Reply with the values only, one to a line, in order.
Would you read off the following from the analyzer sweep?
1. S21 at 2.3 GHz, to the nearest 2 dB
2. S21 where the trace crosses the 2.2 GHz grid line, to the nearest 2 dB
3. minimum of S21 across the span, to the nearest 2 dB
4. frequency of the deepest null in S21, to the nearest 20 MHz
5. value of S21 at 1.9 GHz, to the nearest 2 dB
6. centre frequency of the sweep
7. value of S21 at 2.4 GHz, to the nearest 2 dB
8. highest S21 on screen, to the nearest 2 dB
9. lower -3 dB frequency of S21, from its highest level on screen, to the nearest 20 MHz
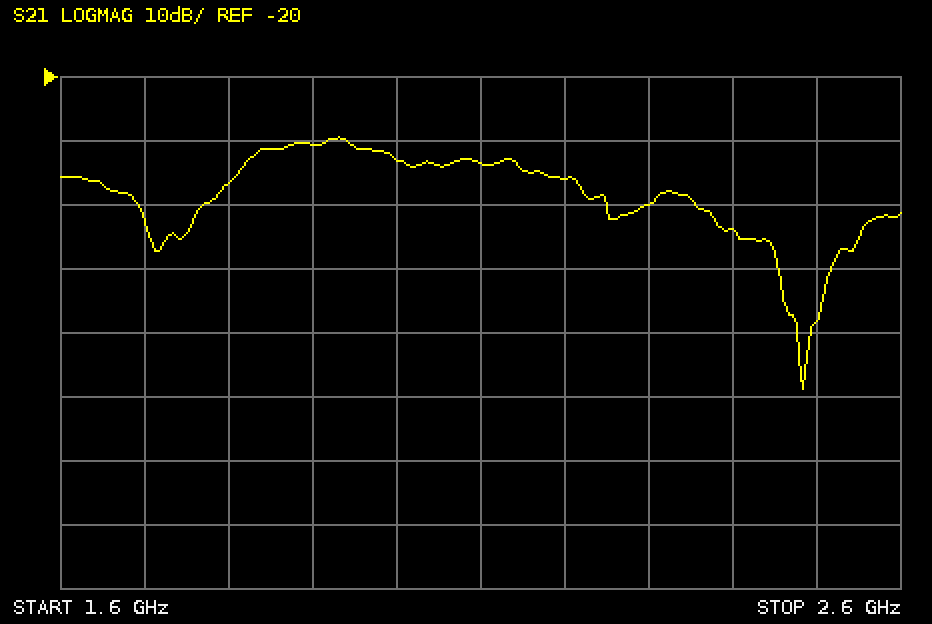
-40 dB
-36 dB
-68 dB
2.48 GHz
-30 dB
2.1 GHz
-44 dB
-30 dB
1.82 GHz
